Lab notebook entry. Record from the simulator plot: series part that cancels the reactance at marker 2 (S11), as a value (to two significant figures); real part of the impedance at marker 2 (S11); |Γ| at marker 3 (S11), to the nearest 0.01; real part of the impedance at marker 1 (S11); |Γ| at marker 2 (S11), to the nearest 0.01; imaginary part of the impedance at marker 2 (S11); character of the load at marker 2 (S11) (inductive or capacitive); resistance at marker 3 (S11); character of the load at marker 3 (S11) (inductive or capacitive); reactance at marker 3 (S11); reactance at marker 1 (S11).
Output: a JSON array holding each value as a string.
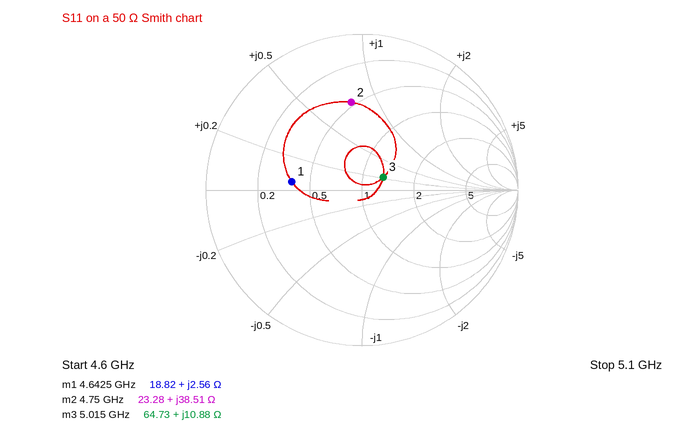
["870 fF", "23.28 Ω", "0.16", "18.82 Ω", "0.57", "+38.51 Ω", "inductive", "64.73 Ω", "inductive", "+10.88 Ω", "+2.56 Ω"]
